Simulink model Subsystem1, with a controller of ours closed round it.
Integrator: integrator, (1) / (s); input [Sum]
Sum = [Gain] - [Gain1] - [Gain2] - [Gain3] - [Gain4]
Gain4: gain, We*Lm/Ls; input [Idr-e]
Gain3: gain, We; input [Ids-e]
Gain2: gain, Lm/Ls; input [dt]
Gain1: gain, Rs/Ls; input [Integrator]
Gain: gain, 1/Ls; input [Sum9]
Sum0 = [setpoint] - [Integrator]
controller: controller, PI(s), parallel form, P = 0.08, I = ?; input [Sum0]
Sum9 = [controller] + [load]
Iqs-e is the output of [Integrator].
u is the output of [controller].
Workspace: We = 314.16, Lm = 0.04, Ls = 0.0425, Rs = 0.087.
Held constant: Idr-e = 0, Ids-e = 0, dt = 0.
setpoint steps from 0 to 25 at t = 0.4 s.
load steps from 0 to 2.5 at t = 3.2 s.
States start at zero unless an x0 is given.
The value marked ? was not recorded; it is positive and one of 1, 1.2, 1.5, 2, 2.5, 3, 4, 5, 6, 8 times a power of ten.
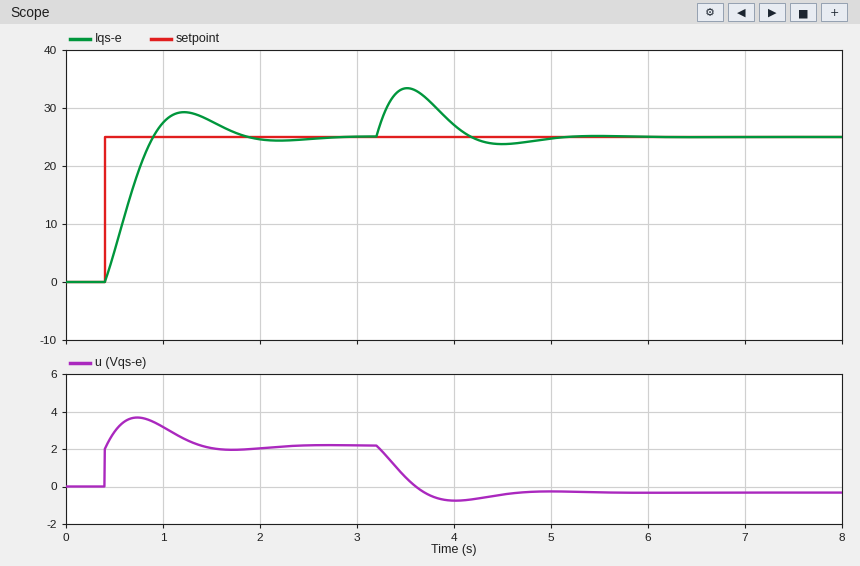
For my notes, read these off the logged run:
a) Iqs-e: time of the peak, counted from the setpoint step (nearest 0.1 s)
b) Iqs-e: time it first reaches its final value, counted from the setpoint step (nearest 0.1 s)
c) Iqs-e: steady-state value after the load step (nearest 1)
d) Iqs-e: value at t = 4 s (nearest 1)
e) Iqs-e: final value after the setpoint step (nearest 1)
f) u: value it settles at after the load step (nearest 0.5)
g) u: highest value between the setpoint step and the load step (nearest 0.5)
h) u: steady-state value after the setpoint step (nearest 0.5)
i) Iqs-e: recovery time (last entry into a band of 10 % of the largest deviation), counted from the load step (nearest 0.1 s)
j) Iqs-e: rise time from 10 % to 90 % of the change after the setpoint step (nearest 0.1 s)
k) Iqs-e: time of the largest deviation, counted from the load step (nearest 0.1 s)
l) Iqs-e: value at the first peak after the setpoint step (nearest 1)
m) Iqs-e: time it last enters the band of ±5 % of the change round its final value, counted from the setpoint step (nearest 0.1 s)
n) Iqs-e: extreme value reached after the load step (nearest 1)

0.8 s
0.5 s
25
27
25
-0.5
3.5
2.0
1.6 s
0.4 s
0.3 s
29
1.3 s
33
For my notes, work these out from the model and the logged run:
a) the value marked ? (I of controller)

0.6
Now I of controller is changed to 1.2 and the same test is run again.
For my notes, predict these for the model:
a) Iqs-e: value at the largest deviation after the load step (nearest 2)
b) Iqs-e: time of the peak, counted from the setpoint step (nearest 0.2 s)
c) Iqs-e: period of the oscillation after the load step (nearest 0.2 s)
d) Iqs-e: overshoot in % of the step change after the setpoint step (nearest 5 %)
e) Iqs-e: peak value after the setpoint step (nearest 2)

32
0.6 s
1.2 s
30 %
32
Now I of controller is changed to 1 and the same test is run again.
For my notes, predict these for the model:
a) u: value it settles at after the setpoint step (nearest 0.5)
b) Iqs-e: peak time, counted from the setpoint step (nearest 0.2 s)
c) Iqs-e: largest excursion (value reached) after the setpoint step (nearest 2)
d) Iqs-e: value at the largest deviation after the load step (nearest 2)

2.0
0.6 s
32
32
